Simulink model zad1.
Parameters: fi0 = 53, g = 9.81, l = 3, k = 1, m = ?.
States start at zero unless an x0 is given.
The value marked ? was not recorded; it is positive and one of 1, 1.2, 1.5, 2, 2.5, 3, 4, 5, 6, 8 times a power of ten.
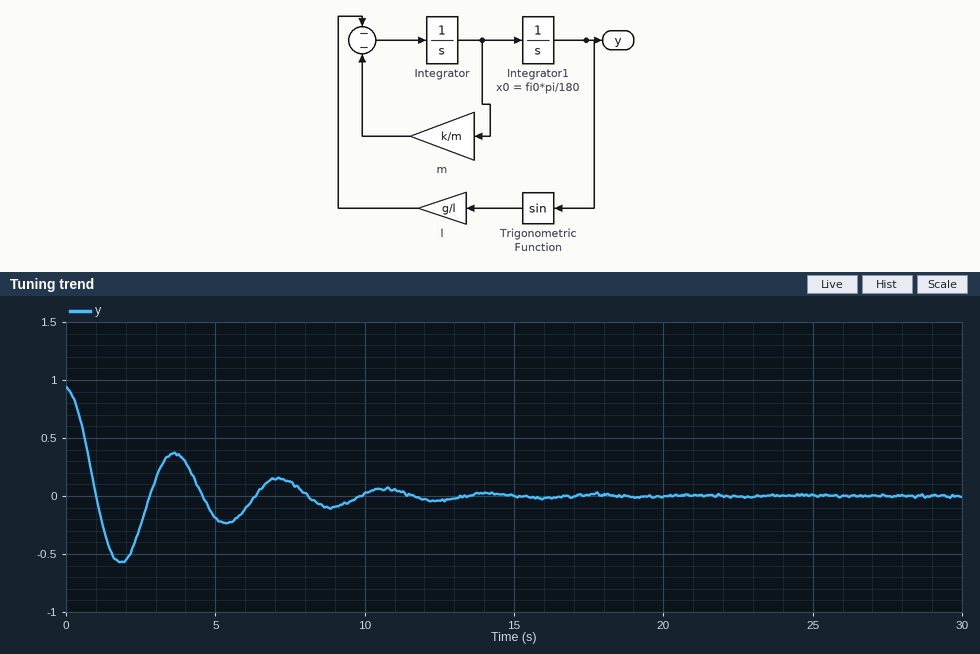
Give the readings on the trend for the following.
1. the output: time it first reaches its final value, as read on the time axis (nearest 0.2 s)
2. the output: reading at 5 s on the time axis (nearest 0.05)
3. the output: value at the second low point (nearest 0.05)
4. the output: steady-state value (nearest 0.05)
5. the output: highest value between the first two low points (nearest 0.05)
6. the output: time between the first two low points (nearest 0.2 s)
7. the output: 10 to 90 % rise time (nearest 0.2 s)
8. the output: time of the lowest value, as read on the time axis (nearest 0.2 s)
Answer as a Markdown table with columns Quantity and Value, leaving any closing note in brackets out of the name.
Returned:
| Quantity | Value |
|---|---|
| the output: time it first reaches its final value, as read on the time axis | 1.0 s |
| the output: reading at 5 s on the time axis | -0.20 |
| the output: value at the second low point | -0.25 |
| the output: steady-state value | 0.00 |
| the output: highest value between the first two low points | 0.35 |
| the output: time between the first two low points | 3.6 s |
| the output: 10 to 90 % rise time | 0.6 s |
| the output: time of the lowest value, as read on the time axis | 1.8 s |
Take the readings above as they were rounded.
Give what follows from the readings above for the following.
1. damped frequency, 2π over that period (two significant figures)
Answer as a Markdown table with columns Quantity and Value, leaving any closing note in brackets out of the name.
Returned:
| Quantity | Value |
|---|---|
| damped frequency, 2π over that period | 1.7 rad/s |
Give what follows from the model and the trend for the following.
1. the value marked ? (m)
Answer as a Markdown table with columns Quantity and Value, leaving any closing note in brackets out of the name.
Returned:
| Quantity | Value |
|---|---|
| the value marked ? | 2 |
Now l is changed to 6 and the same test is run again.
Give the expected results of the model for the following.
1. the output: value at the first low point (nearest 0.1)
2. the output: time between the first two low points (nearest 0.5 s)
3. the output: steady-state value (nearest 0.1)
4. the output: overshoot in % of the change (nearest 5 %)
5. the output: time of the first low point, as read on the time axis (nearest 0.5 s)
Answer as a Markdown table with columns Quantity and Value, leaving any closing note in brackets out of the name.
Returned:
| Quantity | Value |
|---|---|
| the output: value at the first low point | -0.5 |
| the output: time between the first two low points | 5.0 s |
| the output: steady-state value | 0.0 |
| the output: overshoot in % of the change | 50 % |
| the output: time of the first low point, as read on the time axis | 2.5 s |
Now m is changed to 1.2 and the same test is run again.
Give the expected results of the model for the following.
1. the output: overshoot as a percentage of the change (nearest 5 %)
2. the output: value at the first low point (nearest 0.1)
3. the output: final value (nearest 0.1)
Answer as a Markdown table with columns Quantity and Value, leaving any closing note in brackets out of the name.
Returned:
| Quantity | Value |
|---|---|
| the output: overshoot as a percentage of the change | 45 % |
| the output: value at the first low point | -0.4 |
| the output: final value | 0.0 |
